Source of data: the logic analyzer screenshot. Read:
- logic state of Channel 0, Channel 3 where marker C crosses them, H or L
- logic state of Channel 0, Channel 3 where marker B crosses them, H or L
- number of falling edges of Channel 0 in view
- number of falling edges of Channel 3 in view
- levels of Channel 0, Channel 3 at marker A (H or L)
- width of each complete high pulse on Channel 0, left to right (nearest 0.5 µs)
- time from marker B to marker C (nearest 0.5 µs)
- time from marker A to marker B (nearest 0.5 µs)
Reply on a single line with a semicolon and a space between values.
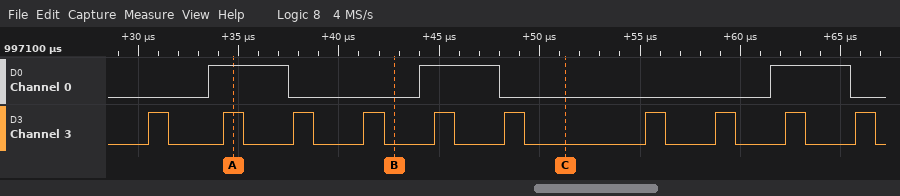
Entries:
Channel 0=L, Channel 3=L; Channel 0=L, Channel 3=L; 3; 10; Channel 0=H, Channel 3=H; 4 µs, 4 µs, 4 µs; 8.5 µs; 8 µs
